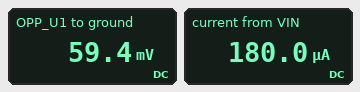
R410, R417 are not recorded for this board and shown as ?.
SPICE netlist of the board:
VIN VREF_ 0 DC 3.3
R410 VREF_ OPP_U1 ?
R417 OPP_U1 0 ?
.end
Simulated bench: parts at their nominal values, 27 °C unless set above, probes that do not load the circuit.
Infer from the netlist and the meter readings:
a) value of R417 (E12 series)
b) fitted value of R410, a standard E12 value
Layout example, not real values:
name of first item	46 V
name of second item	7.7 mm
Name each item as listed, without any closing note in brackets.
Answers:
value of R417	330 Ω
fitted value of R410, a standard E12 value	18 kΩ
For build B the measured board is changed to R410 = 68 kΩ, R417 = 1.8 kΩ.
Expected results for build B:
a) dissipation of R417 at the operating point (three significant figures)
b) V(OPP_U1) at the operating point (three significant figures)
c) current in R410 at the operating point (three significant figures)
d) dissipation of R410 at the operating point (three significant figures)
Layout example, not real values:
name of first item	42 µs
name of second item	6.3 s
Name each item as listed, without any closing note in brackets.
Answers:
dissipation of R417 at the operating point	4.02 µW
V(OPP_U1) at the operating point	85.1 mV
current in R410 at the operating point	47.3 µA
dissipation of R410 at the operating point	152 µW
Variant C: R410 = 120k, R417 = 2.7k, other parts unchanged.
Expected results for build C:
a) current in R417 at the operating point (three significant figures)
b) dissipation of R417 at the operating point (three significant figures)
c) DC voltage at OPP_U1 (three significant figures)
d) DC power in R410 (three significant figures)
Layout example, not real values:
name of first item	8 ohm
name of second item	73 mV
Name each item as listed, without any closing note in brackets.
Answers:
current in R417 at the operating point	26.9 µA
dissipation of R417 at the operating point	1.95 µW
DC voltage at OPP_U1	72.6 mV
DC power in R410	86.8 µW
